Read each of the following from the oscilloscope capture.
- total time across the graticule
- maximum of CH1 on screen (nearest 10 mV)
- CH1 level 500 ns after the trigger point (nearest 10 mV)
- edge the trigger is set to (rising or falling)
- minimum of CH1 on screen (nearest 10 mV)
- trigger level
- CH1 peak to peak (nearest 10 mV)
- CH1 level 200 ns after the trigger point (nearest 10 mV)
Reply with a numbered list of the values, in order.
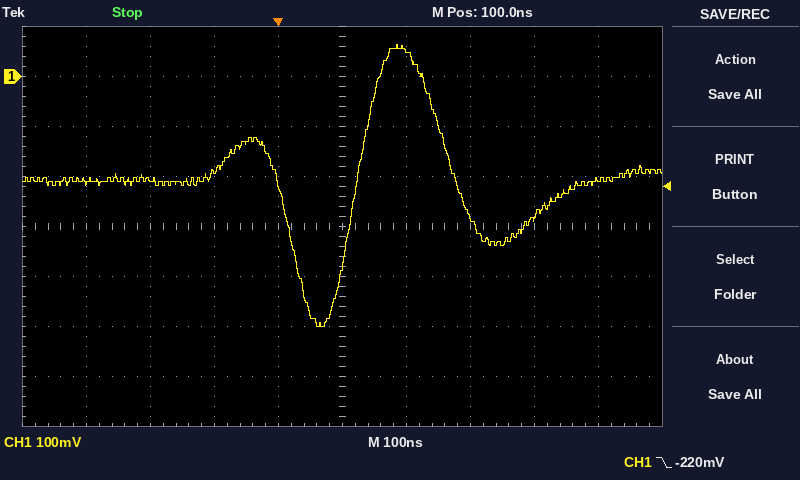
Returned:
1. 1 µs
2. 60 mV
3. -210 mV
4. falling
5. -500 mV
6. -220 mV
7. 560 mV
8. 50 mV
